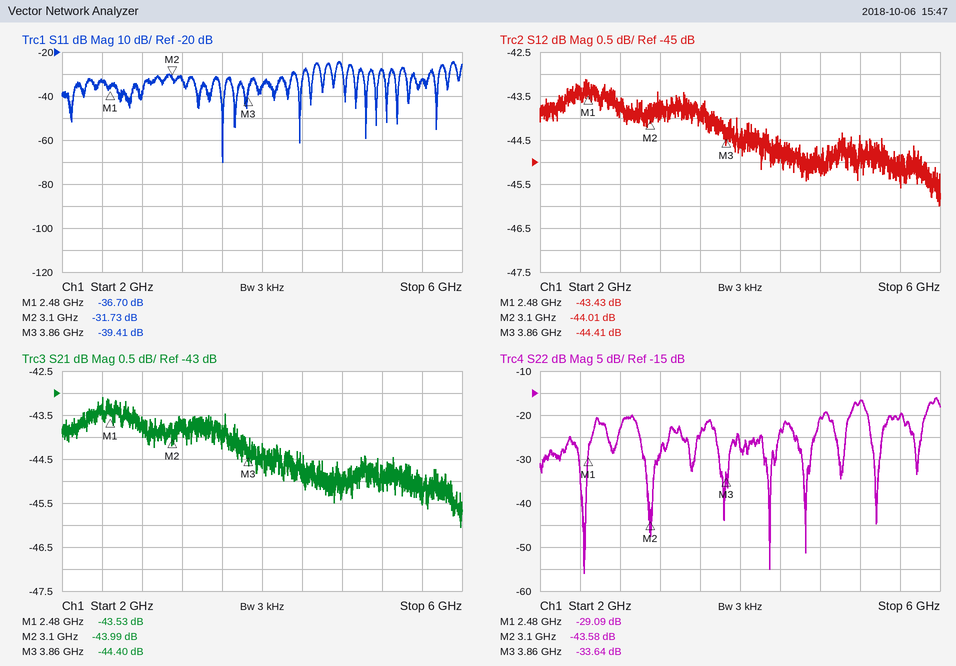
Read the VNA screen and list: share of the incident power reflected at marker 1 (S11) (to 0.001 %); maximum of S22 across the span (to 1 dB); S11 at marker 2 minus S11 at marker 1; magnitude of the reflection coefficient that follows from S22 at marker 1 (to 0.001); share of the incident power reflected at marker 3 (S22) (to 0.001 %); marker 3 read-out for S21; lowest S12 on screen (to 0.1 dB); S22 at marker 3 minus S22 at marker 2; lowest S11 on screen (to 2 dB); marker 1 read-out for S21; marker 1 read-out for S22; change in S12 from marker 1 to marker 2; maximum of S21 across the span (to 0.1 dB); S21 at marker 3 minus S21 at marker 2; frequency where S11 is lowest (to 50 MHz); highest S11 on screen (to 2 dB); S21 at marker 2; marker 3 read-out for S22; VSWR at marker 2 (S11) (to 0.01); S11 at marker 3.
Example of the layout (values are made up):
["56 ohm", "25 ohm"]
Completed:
["0.021 %", "-16 dB", "4.97 dB", "0.035", "0.043 %", "-44.40 dB", "-46.0 dB", "9.94 dB", "-70 dB", "-43.53 dB", "-29.09 dB", "-0.58 dB", "-43.1 dB", "-0.41 dB", "3.60 GHz", "-24 dB", "-43.99 dB", "-33.64 dB", "1.05", "-39.41 dB"]
